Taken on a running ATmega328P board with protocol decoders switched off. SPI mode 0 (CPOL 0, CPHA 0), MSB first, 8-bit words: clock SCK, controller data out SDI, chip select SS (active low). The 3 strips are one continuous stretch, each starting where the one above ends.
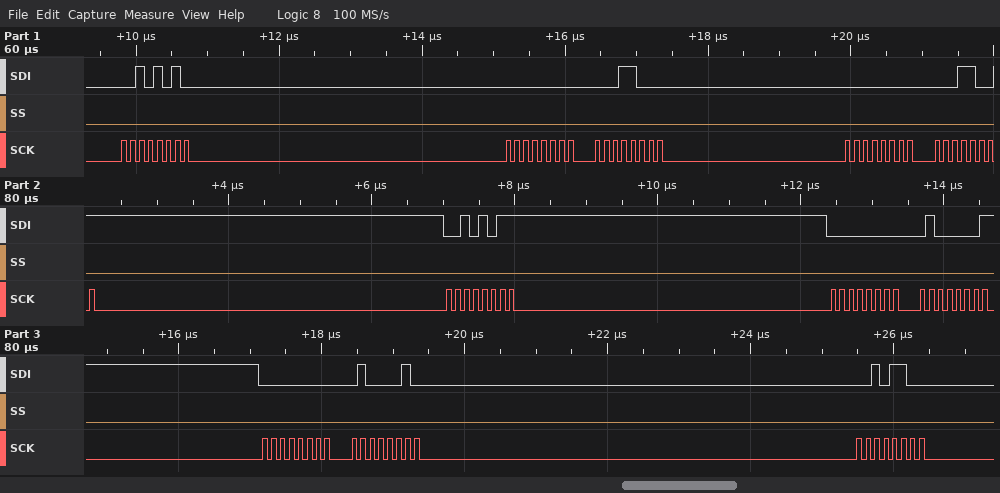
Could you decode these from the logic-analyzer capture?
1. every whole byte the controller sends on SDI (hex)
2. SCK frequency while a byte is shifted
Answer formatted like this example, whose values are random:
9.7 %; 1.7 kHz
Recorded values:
2A 00 18 00 19 2B 00 41 00 42 2C; 8 MHz
